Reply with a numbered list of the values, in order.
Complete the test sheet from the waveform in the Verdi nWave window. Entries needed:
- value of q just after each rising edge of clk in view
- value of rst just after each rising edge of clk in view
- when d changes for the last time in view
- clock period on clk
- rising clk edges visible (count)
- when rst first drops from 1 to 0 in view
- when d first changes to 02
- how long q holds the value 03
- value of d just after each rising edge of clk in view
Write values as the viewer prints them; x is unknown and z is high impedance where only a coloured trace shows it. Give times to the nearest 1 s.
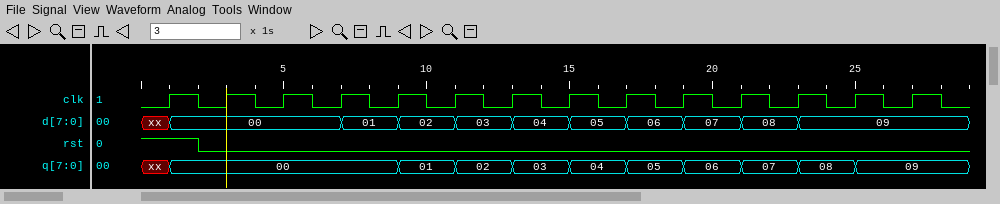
1. 00, 00, 00, 00, 01, 02, 03, 04, 05, 06, 07, 08, 09, 09
2. 1 0 0 0 0 0 0 0 0 0 0 0 0 0
3. 23 s
4. 2 s
5. 14
6. 2 s
7. 9 s
8. 2 s
9. 00, 00, 00, 01, 02, 03, 04, 05, 06, 07, 08, 09, 09, 09
